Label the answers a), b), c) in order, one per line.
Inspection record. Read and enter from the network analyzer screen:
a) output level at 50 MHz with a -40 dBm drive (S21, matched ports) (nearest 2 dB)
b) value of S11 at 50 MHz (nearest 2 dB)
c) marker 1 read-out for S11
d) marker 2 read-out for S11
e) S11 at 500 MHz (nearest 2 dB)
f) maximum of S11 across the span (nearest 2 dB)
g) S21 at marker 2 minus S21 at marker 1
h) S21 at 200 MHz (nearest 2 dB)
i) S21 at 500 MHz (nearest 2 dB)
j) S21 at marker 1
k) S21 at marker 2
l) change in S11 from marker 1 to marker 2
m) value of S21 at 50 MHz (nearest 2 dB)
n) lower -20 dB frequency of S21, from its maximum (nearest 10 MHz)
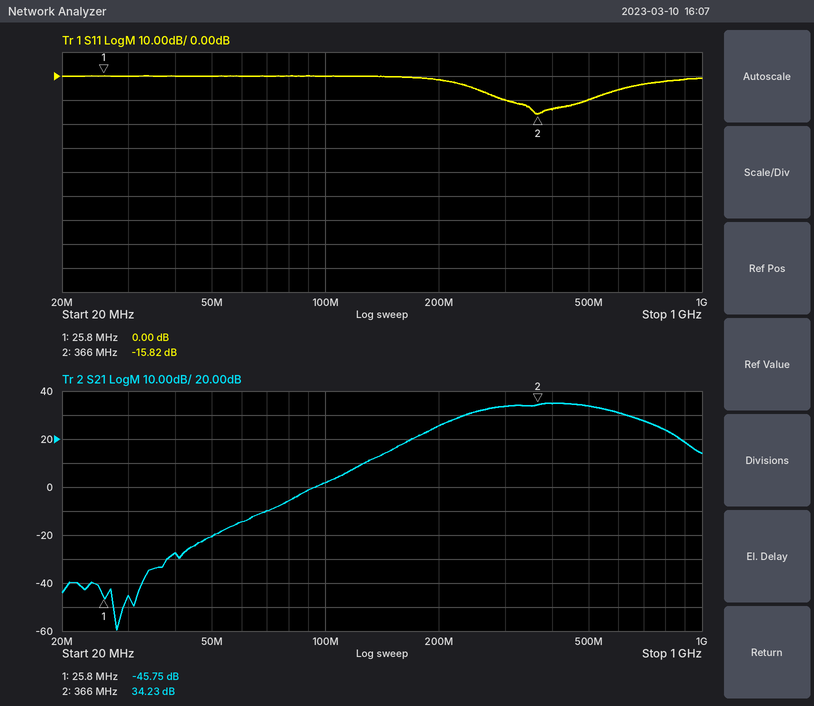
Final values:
a) -60 dBm
b) 0 dB
c) 0.00 dB
d) -15.82 dB
e) -10 dB
f) 0 dB
g) 79.98 dB
h) 26 dB
i) 34 dB
j) -45.75 dB
k) 34.23 dB
l) -15.82 dB
m) -20 dB
n) 150 MHz
